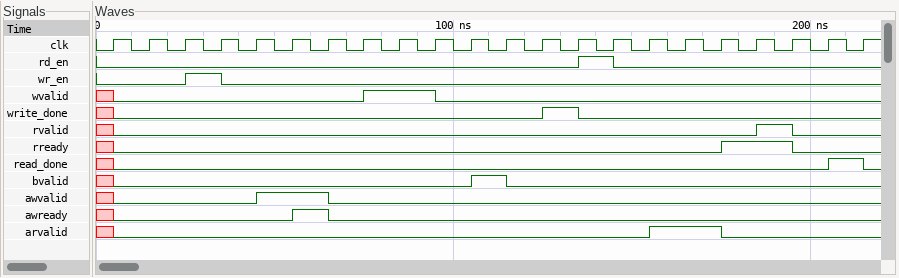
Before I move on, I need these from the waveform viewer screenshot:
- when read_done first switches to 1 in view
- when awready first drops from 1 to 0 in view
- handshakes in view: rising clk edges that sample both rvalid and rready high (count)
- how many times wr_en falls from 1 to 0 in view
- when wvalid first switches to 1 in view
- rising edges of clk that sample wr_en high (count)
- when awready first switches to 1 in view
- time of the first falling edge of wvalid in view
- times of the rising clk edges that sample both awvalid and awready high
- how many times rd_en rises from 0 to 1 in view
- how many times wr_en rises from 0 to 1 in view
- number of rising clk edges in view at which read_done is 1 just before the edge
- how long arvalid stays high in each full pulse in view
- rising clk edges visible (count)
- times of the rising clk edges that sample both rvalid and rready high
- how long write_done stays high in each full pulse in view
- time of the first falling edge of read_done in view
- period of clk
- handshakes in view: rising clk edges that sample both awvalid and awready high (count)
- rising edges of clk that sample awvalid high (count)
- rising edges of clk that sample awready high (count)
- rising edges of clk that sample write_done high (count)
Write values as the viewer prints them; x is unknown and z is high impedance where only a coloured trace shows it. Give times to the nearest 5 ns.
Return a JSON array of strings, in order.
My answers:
["205 ns", "65 ns", "1", "1", "75 ns", "1", "55 ns", "95 ns", "65 ns", "1", "1", "1", "20 ns", "22", "195 ns", "10 ns", "215 ns", "10 ns", "1", "2", "1", "1"]
